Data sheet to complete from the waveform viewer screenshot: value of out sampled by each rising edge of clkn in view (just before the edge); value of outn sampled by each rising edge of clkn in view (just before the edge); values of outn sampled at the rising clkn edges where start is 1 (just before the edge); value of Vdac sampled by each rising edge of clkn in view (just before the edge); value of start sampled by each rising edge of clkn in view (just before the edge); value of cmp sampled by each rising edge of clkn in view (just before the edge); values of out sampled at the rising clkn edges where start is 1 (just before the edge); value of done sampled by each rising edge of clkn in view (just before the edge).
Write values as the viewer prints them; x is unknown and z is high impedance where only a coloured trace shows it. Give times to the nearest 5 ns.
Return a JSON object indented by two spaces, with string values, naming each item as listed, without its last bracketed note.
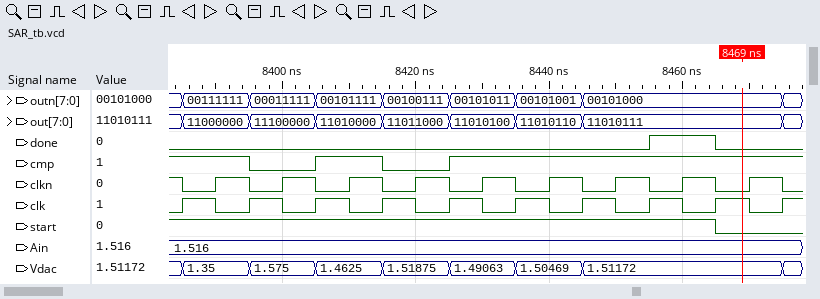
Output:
{
  "value of out sampled by each rising edge of clkn in view": "11000000, 11100000, 11010000, 11011000, 11010100, 11010110, 11010111, 11010111, 11010111",
  "value of outn sampled by each rising edge of clkn in view": "00111111, 00011111, 00101111, 00100111, 00101011, 00101001, 00101000, 00101000, 00101000",
  "values of outn sampled at the rising clkn edges where start is 1": "00111111, 00011111, 00101111, 00100111, 00101011, 00101001, 00101000, 00101000",
  "value of Vdac sampled by each rising edge of clkn in view": "1.35, 1.575, 1.4625, 1.51875, 1.49063, 1.50469, 1.51172, 1.51172, 1.51172",
  "value of start sampled by each rising edge of clkn in view": "1 1 1 1 1 1 1 1 0",
  "value of cmp sampled by each rising edge of clkn in view": "1 0 1 0 1 1 1 1 1",
  "values of out sampled at the rising clkn edges where start is 1": "11000000, 11100000, 11010000, 11011000, 11010100, 11010110, 11010111, 11010111",
  "value of done sampled by each rising edge of clkn in view": "0 0 0 0 0 0 0 1 0"
}
